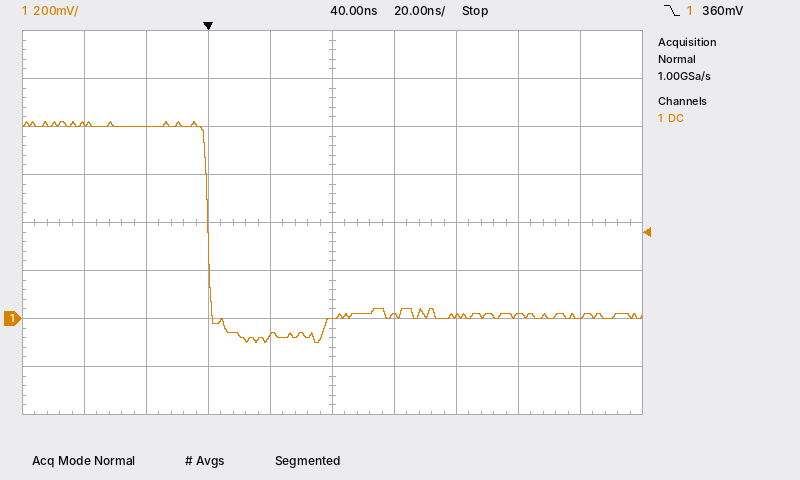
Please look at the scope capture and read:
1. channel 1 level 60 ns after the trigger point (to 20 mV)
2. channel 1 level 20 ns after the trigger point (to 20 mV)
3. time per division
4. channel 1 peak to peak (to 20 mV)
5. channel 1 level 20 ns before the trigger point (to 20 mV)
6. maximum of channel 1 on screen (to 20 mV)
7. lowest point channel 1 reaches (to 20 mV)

20 mV
-80 mV
20 ns
920 mV
800 mV
820 mV
-100 mV
